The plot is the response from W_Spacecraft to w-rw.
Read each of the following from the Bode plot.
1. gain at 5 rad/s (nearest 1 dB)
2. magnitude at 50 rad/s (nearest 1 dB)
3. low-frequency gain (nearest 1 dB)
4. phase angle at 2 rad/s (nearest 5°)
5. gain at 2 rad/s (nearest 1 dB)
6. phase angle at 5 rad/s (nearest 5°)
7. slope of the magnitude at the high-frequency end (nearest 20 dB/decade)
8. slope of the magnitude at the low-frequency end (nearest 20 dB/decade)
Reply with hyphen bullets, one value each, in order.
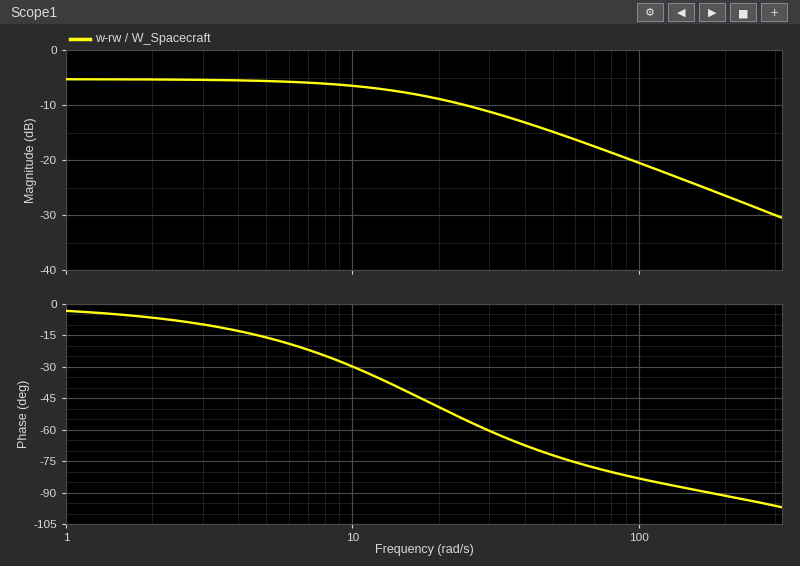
- -6 dB
- -15 dB
- -5 dB
- -5°
- -5 dB
- -15°
- -20 dB/decade
- 0 dB/decade
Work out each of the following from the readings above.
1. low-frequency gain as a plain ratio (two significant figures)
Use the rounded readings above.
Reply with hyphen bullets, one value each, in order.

- 0.56
